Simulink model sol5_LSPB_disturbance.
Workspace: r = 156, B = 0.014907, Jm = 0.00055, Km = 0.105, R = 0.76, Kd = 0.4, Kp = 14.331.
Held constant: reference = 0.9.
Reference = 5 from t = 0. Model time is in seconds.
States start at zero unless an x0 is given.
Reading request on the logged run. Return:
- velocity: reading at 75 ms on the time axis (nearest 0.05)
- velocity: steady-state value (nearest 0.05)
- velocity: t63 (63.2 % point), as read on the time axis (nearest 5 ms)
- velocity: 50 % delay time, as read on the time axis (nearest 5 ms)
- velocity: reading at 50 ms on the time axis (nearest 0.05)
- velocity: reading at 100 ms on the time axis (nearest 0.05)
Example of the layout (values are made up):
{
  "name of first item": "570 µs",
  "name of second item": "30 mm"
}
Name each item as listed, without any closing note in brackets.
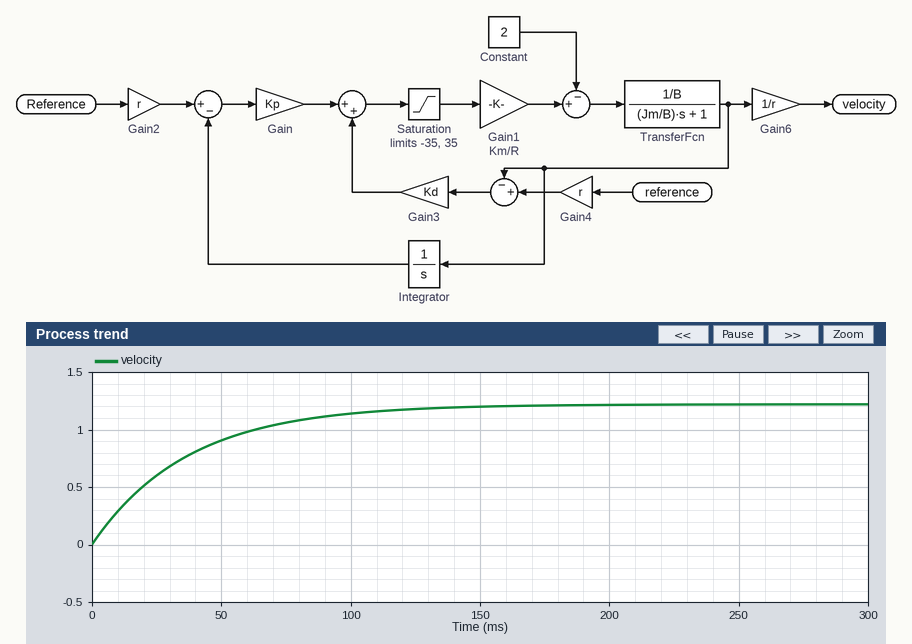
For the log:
{
  "velocity: reading at 75 ms on the time axis": "1.05",
  "velocity: steady-state value": "1.20",
  "velocity: t63 (63.2 % point), as read on the time axis": "35 ms",
  "velocity: 50 % delay time, as read on the time axis": "25 ms",
  "velocity: reading at 50 ms on the time axis": "0.90",
  "velocity: reading at 100 ms on the time axis": "1.15"
}
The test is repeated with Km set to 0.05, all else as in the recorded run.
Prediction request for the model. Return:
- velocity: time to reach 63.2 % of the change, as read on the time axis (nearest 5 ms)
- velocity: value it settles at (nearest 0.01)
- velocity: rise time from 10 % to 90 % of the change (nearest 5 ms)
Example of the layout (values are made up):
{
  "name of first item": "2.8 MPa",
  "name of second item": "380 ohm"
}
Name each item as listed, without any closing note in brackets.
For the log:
{
  "velocity: time to reach 63.2 % of the change, as read on the time axis": "35 ms",
  "velocity: value it settles at": "0.13",
  "velocity: rise time from 10 % to 90 % of the change": "80 ms"
}
